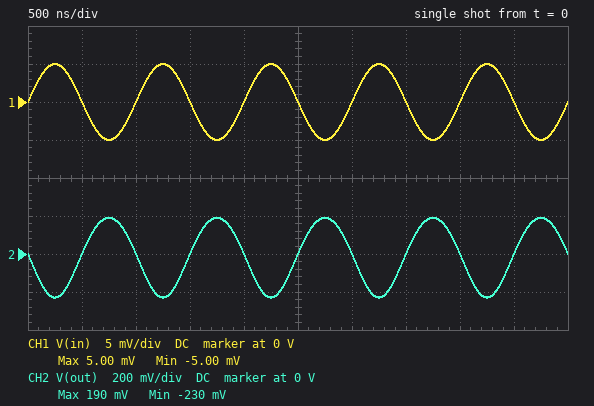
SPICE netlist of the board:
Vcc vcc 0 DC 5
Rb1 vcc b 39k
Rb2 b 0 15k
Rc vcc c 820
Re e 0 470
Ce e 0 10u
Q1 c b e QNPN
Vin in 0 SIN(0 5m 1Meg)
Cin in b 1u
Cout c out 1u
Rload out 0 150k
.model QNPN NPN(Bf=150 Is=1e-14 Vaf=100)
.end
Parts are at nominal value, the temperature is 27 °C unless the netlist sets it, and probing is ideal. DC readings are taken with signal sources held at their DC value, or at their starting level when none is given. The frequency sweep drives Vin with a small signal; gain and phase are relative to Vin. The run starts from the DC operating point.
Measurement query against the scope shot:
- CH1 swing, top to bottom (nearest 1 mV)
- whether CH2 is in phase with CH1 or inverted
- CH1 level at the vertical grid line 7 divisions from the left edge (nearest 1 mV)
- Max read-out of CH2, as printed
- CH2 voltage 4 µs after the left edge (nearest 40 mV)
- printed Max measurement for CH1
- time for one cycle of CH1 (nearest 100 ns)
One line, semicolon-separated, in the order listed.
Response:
10 mV; inverted; 0 V; 190 mV; 0 V; 5.00 mV; 1.0 µs
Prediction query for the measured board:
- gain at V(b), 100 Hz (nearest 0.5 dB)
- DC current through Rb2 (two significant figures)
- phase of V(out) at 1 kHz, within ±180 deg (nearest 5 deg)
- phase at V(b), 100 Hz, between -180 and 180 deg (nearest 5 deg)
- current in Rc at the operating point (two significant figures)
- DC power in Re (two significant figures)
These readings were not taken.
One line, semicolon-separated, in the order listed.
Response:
-0.5 dB; 86 µA; -140 deg; 10 deg; 1.3 mA; 850 µW
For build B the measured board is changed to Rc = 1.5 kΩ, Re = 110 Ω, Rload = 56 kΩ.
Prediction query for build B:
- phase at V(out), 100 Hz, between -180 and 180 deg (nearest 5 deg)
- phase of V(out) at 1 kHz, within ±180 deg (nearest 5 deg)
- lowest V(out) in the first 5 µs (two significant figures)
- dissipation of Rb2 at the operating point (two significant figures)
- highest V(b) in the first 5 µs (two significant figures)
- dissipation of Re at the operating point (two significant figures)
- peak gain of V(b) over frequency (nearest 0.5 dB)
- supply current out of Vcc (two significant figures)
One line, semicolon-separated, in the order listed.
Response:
-90 deg; -100 deg; -76 mV; 69 µW; 1.0 V; 1.0 mW; 0 dB; 3.1 mA
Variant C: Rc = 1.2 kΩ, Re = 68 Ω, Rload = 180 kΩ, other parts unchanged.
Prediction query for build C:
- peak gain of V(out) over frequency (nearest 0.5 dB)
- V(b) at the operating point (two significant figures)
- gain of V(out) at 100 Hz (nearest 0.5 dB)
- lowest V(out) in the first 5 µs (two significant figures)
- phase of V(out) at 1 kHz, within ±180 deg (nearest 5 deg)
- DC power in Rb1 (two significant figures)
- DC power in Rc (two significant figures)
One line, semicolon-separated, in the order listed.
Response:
37.5 dB; 950 mV; -0.5 dB; -80 mV; -100 deg; 420 µW; 18 mW
